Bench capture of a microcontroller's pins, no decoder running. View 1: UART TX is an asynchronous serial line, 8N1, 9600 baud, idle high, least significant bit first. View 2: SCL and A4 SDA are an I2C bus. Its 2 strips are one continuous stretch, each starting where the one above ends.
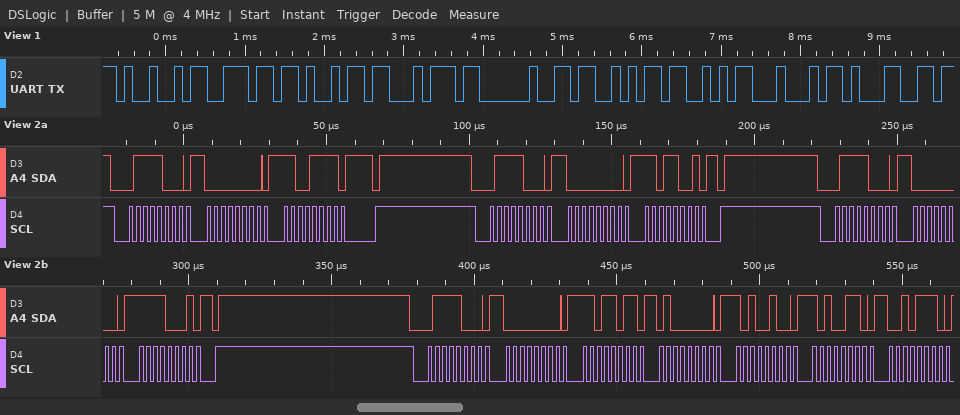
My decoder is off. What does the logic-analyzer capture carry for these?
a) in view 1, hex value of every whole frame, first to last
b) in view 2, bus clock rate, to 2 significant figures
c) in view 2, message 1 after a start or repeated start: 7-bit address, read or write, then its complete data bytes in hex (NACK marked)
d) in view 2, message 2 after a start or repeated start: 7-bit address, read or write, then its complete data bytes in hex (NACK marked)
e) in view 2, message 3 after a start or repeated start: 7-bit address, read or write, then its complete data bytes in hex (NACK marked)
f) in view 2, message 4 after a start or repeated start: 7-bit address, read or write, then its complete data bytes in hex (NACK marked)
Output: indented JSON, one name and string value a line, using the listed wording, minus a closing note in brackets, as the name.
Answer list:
{
  "in view 1, hex value of every whole frame, first to last": "49 6E 69 74 20 53 53 44 31",
  "in view 2, bus clock rate, to 2 significant figures": "400 kHz",
  "in view 2, message 1 after a start or repeated start: 7-bit address, read or write, then its complete data bytes in hex": "0x3C write: 00 CF",
  "in view 2, message 2 after a start or repeated start: 7-bit address, read or write, then its complete data bytes in hex": "0x3C write: 00 D9",
  "in view 2, message 3 after a start or repeated start: 7-bit address, read or write, then its complete data bytes in hex": "0x3C write: 00 F1",
  "in view 2, message 4 after a start or repeated start: 7-bit address, read or write, then its complete data bytes in hex": "0x3C write: 00 DB 40 A4 A6 2E"
}
